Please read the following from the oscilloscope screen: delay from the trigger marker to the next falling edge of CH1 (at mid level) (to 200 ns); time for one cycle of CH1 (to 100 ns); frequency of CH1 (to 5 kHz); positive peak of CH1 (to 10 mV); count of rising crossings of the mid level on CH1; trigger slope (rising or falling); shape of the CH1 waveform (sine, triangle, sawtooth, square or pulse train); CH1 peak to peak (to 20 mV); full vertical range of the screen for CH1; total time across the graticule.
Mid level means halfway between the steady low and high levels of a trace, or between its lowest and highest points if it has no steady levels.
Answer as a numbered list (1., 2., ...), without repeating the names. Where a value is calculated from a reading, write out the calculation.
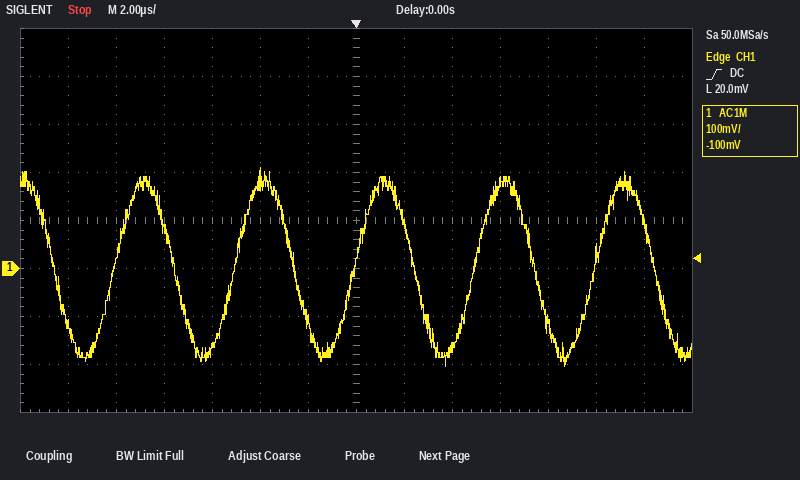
1. 2.4 µs
2. 5.0 µs
3. 1 / 5.0 µs ≈ 200 kHz
4. 210 mV
5. 5
6. rising
7. sine
8. 420 mV
9. 800 mV
10. 28 µs
